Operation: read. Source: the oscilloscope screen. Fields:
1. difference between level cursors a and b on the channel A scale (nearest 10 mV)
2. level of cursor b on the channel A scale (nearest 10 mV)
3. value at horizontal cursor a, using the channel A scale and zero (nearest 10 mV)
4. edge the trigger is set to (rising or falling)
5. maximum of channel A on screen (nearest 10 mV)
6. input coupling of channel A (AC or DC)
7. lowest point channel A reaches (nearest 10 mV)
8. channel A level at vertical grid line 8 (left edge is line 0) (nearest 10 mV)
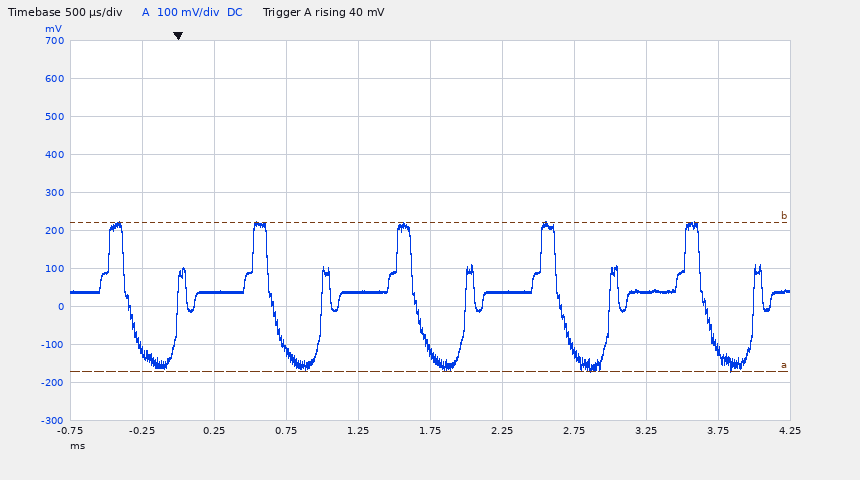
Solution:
390 mV
220 mV
-170 mV
rising
220 mV
DC
-170 mV
40 mV
